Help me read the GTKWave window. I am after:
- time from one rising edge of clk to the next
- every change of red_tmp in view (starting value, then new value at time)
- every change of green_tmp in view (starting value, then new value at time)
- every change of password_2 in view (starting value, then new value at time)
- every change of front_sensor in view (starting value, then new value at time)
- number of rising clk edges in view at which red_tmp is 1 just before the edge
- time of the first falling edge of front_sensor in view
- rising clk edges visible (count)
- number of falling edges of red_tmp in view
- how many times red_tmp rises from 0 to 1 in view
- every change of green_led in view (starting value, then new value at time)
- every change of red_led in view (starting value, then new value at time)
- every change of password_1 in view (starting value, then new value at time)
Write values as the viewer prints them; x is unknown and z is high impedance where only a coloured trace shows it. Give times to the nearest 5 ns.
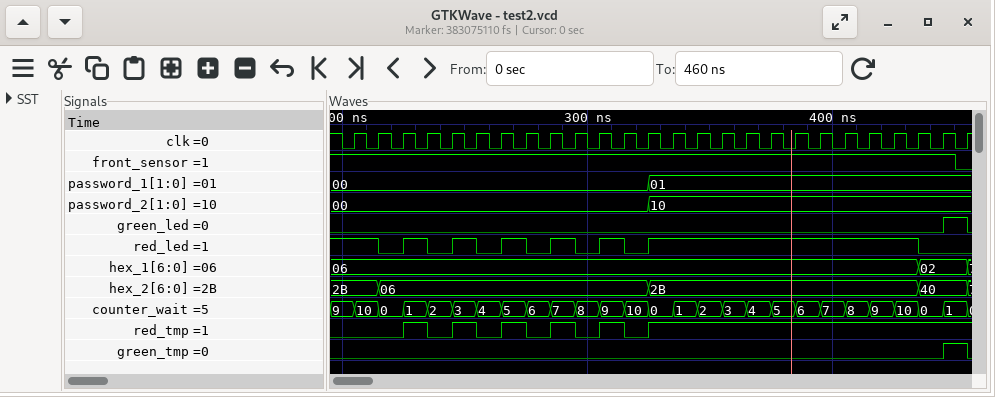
10 ns
0, 1 at 225 ns, 0 at 235 ns, 1 at 245 ns, 0 at 255 ns, 1 at 265 ns, 0 at 275 ns, 1 at 285 ns, 0 at 295 ns, 1 at 305 ns, 0 at 315 ns, 1 at 325 ns
0, 1 at 445 ns, 0 at 455 ns
00, 10 at 325 ns
1, 0 at 450 ns
18
450 ns
26
5
6
0, 1 at 445 ns, 0 at 455 ns
1, 0 at 215 ns, 1 at 225 ns, 0 at 235 ns, 1 at 245 ns, 0 at 255 ns, 1 at 265 ns, 0 at 275 ns, 1 at 285 ns, 0 at 295 ns, 1 at 305 ns, 0 at 315 ns, 1 at 325 ns, 0 at 435 ns
00, 01 at 325 ns
